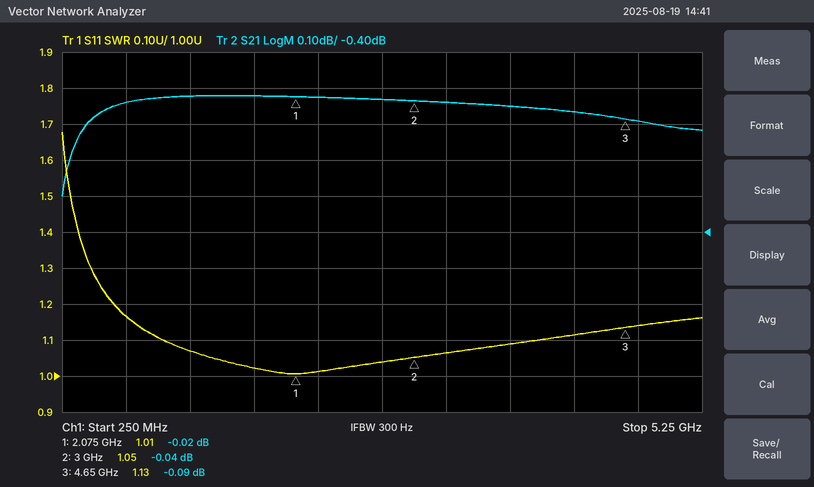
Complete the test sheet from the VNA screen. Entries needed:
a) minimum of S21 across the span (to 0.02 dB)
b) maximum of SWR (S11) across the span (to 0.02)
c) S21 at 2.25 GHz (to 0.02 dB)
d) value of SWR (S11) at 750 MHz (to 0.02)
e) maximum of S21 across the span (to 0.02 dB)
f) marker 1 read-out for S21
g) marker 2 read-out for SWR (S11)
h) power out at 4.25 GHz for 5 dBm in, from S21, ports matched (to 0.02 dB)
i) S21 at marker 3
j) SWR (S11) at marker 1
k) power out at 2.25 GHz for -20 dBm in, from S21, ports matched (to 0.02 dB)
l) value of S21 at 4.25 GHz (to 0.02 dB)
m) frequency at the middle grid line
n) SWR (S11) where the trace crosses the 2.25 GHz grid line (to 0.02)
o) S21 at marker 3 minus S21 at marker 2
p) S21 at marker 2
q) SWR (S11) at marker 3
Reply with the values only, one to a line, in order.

-0.30 dB
1.68
-0.02 dB
1.16
-0.02 dB
-0.02 dB
1.05
4.94 dBm
-0.09 dB
1.01
-20.02 dBm
-0.06 dB
2.75 GHz
1.02
-0.05 dB
-0.04 dB
1.13
